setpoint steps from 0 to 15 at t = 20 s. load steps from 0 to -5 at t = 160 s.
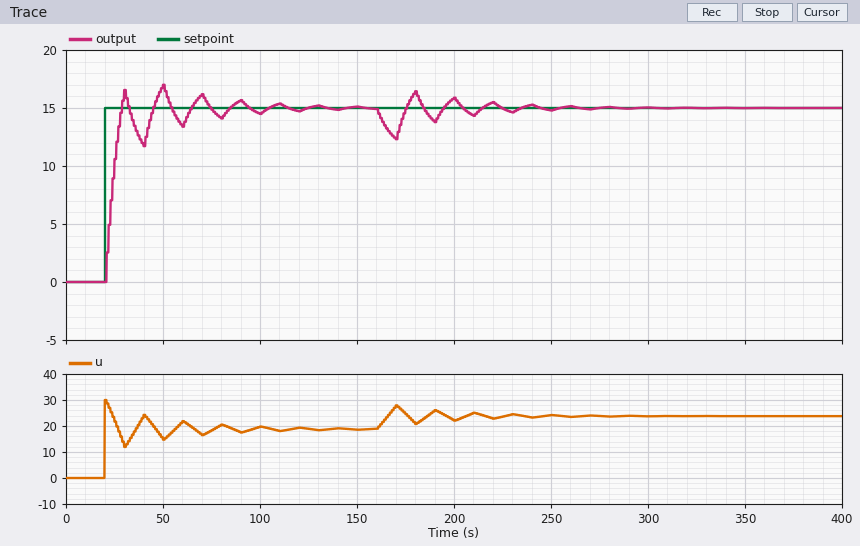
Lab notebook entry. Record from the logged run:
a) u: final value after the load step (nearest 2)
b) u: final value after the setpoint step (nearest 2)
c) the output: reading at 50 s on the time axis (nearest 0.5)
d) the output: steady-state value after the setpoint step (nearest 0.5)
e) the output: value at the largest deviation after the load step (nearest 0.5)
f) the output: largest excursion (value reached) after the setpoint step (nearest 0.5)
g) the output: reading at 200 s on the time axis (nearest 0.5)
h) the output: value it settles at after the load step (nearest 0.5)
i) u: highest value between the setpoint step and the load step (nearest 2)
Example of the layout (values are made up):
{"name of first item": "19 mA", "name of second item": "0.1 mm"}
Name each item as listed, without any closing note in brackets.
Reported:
{"u: final value after the load step": "24", "u: final value after the setpoint step": "18", "the output: reading at 50 s on the time axis": "17.0", "the output: steady-state value after the setpoint step": "15.0", "the output: value at the largest deviation after the load step": "12.5", "the output: largest excursion (value reached) after the setpoint step": "17.0", "the output: reading at 200 s on the time axis": "16.0", "the output: value it settles at after the load step": "15.0", "u: highest value between the setpoint step and the load step": "30"}
